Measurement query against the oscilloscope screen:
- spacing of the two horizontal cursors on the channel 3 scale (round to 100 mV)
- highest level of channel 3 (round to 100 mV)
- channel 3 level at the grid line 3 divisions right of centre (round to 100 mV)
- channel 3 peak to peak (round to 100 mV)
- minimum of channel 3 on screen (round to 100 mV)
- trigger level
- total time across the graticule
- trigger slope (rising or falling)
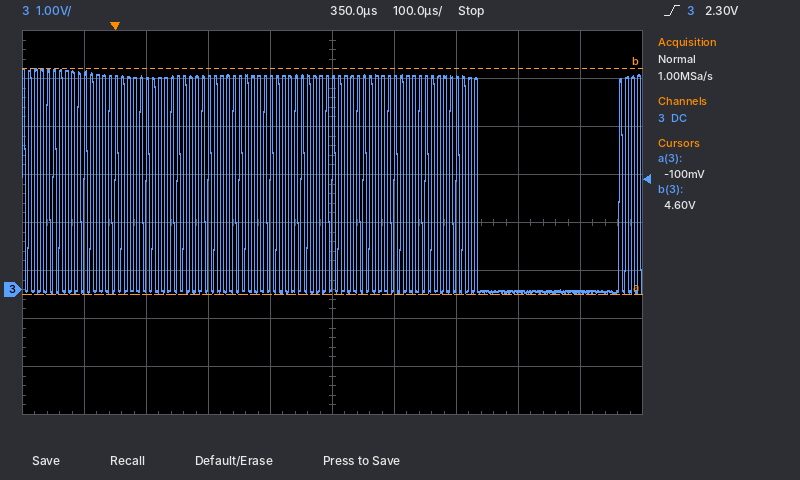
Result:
4.7 V
4.6 V
0.0 V
4.7 V
-100 mV
2.30 V
1 ms
rising
